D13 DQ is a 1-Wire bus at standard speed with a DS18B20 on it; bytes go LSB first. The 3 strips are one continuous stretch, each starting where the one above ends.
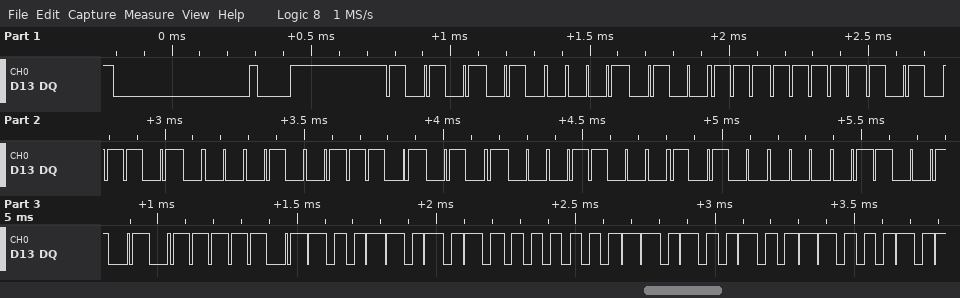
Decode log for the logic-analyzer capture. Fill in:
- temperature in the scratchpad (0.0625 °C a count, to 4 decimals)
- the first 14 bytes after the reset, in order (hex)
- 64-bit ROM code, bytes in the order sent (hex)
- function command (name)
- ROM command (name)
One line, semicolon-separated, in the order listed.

21.5625 °C; 55 28 FF B5 90 AB 18 05 A6 BE 59 01 4B 46; 28 FF B5 90 AB 18 05 A6; Read Scratchpad; Match ROM
